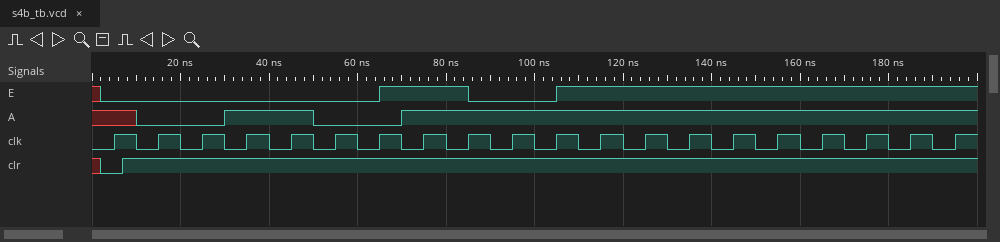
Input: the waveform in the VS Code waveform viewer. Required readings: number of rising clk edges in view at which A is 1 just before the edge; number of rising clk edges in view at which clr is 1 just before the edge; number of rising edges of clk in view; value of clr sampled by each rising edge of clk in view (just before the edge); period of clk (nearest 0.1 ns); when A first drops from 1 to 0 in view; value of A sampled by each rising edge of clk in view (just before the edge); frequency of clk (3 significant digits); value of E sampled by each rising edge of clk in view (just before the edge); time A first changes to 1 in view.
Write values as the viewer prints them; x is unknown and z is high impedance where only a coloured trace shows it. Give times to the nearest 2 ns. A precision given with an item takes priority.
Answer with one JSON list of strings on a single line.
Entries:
["15", "19", "20", "0 1 1 1 1 1 1 1 1 1 1 1 1 1 1 1 1 1 1 1", "10 ns", "50 ns", "x 0 0 1 1 0 0 1 1 1 1 1 1 1 1 1 1 1 1 1", "100 MHz", "0 0 0 0 0 0 0 1 1 0 0 1 1 1 1 1 1 1 1 1", "30 ns"]
